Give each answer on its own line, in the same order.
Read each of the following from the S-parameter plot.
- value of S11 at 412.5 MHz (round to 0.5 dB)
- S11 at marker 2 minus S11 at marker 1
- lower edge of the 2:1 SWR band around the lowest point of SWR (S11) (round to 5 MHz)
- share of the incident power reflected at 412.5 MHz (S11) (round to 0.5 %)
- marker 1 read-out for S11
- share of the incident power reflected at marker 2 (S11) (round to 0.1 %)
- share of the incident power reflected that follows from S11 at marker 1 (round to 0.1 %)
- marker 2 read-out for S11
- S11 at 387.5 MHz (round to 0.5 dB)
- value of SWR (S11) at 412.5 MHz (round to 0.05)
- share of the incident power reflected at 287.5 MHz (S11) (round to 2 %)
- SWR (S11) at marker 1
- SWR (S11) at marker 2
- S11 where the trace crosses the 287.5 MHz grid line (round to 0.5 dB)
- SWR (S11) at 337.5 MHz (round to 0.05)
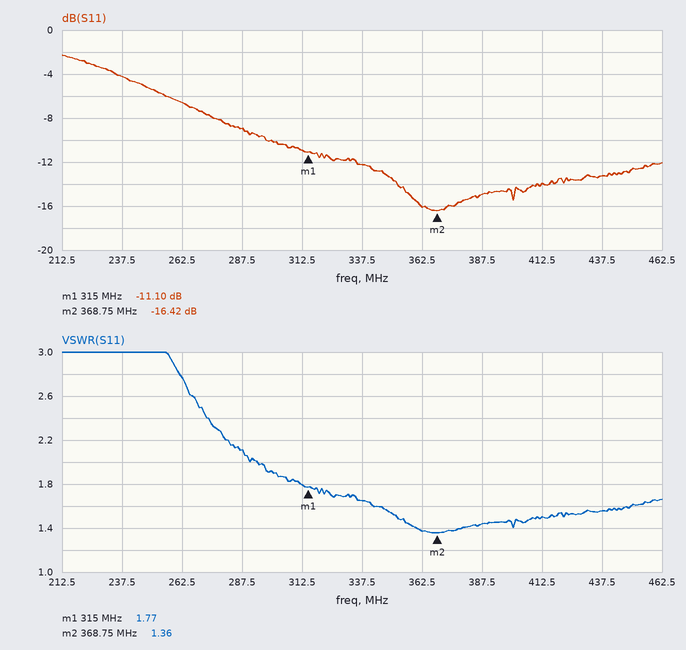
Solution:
-14.0 dB
-5.32 dB
295 MHz
4.0 %
-11.10 dB
2.3 %
7.8 %
-16.42 dB
-15.0 dB
1.50
12 %
1.77
1.36
-9.0 dB
1.65
